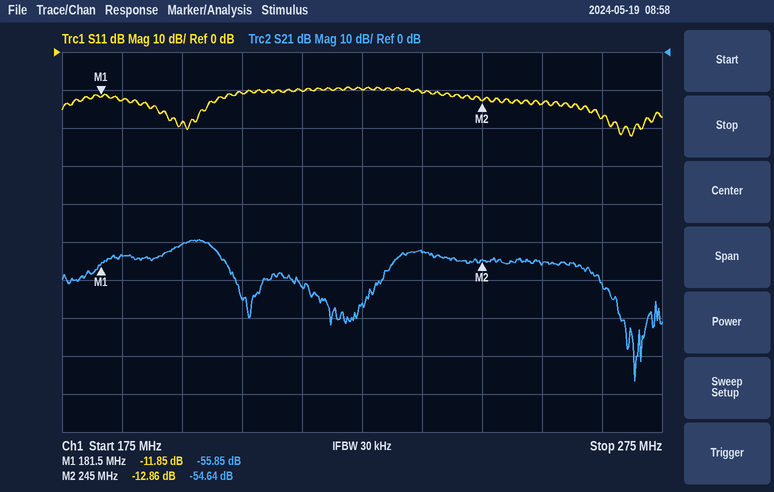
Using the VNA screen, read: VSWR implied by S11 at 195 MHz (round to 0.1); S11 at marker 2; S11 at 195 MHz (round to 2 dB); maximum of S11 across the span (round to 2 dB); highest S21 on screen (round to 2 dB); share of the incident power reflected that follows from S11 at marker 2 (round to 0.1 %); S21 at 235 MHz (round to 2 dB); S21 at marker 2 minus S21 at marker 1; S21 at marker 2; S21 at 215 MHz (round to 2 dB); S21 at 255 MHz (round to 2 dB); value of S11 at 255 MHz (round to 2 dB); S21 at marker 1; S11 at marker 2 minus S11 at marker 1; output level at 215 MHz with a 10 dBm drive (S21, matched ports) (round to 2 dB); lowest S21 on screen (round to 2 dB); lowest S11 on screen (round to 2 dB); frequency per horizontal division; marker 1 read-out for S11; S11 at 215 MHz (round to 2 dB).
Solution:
1.3
-12.86 dB
-18 dB
-10 dB
-50 dB
5.2 %
-52 dB
1.21 dB
-54.64 dB
-62 dB
-56 dB
-14 dB
-55.85 dB
-1.01 dB
-52 dBm
-86 dB
-22 dB
10 MHz
-11.85 dB
-10 dB
